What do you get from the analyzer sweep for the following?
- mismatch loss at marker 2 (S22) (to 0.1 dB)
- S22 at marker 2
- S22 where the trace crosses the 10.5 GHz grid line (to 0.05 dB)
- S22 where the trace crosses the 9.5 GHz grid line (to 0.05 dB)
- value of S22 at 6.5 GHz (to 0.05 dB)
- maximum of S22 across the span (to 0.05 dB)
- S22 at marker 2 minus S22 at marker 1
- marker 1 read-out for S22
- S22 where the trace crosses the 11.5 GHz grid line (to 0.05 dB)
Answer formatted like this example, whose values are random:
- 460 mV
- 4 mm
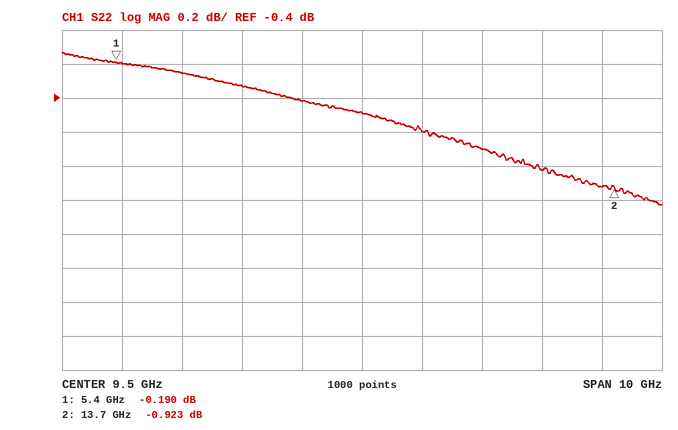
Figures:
- 7.2 dB
- -0.923 dB
- -0.60 dB
- -0.50 dB
- -0.25 dB
- -0.15 dB
- -0.733 dB
- -0.190 dB
- -0.70 dB
